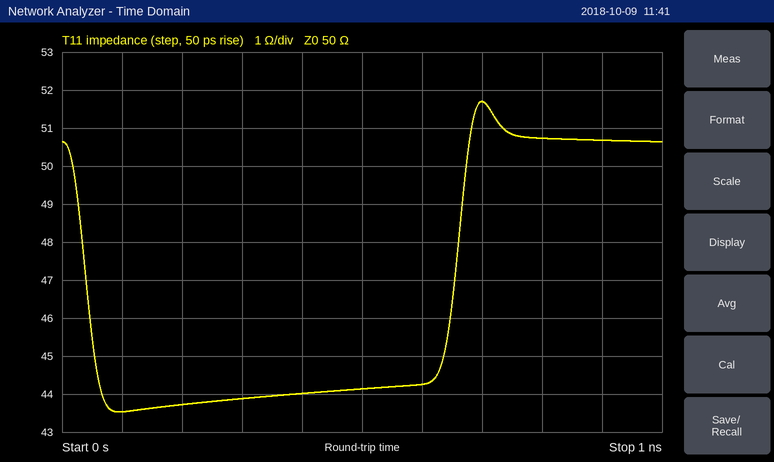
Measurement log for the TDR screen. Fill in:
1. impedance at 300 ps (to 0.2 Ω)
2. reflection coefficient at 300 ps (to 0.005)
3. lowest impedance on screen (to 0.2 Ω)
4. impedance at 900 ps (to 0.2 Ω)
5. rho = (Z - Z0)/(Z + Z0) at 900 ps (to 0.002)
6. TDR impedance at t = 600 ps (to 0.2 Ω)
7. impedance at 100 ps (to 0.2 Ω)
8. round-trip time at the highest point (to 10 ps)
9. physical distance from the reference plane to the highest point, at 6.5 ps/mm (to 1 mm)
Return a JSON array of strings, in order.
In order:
["43.8 Ω", "-0.065", "43.6 Ω", "50.6 Ω", "+0.006", "44.2 Ω", "43.6 Ω", "700 ps", "54 mm"]
